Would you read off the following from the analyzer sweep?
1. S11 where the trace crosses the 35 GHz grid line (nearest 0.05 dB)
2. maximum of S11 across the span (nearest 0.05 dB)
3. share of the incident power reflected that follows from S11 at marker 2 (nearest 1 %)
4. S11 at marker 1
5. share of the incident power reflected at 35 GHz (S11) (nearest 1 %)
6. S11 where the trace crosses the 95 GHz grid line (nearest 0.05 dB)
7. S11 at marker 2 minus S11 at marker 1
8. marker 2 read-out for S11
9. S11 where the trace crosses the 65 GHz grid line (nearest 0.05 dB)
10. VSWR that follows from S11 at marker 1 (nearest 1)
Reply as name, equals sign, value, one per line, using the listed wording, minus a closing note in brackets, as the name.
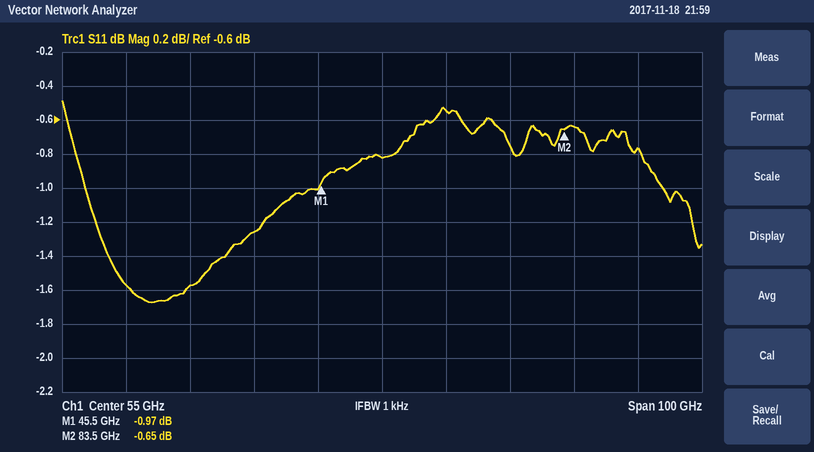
S11 where the trace crosses the 35 GHz grid line = -1.25 dB
maximum of S11 across the span = -0.50 dB
share of the incident power reflected that follows from S11 at marker 2 = 86 %
S11 at marker 1 = -0.97 dB
share of the incident power reflected at 35 GHz (S11) = 75 %
S11 where the trace crosses the 95 GHz grid line = -0.75 dB
S11 at marker 2 minus S11 at marker 1 = 0.32 dB
marker 2 read-out for S11 = -0.65 dB
S11 where the trace crosses the 65 GHz grid line = -0.55 dB
VSWR that follows from S11 at marker 1 = 18
